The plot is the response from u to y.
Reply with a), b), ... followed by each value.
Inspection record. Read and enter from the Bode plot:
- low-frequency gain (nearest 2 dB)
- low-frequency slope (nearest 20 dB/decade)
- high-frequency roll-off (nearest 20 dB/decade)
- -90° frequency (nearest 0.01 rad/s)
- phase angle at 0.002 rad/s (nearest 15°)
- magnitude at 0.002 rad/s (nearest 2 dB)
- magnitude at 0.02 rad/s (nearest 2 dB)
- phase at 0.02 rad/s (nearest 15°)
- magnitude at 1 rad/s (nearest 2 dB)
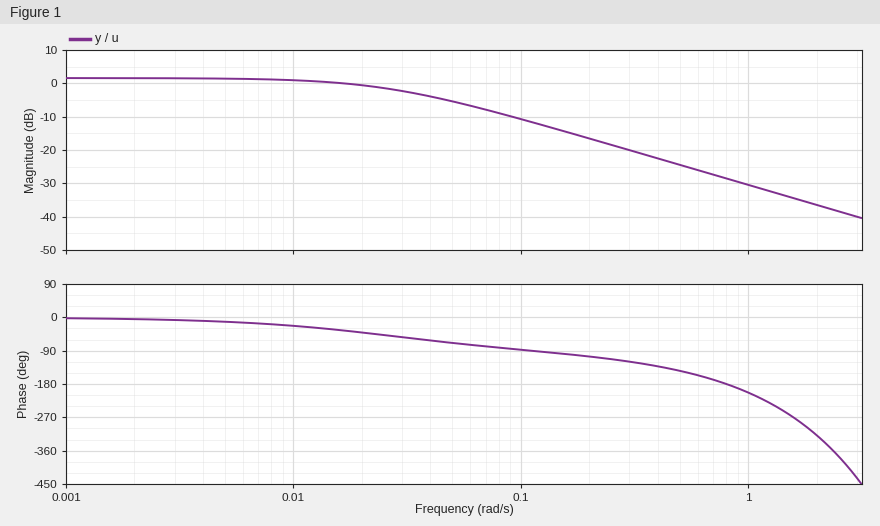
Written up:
a) 2 dB
b) 0 dB/decade
c) -20 dB/decade
d) 0.11 rad/s
e) 0°
f) 2 dB
g) 0 dB
h) -45°
i) -30 dB
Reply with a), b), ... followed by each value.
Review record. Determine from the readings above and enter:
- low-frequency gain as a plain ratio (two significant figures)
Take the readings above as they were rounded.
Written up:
a) 1.3
